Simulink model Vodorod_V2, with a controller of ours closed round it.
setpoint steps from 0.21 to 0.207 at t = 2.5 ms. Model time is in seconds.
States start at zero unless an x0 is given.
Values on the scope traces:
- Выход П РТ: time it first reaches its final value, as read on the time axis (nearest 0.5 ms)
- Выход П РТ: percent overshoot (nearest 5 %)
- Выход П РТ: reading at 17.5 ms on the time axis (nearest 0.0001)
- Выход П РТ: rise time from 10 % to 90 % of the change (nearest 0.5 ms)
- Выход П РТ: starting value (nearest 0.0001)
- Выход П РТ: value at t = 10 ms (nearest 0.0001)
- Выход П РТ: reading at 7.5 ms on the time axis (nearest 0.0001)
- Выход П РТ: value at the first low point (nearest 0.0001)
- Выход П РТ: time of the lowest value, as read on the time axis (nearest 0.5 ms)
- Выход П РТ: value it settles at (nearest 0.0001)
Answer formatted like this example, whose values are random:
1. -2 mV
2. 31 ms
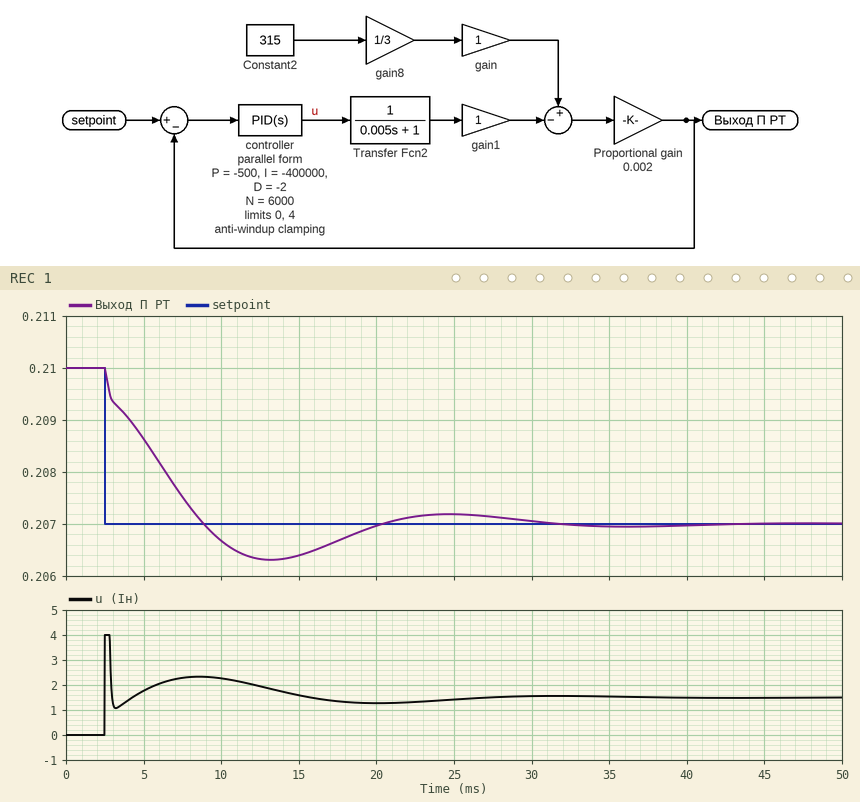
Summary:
1. 9.0 ms
2. 25 %
3. 0.2067
4. 5.5 ms
5. 0.2100
6. 0.2067
7. 0.2075
8. 0.2063
9. 13.0 ms
10. 0.2070
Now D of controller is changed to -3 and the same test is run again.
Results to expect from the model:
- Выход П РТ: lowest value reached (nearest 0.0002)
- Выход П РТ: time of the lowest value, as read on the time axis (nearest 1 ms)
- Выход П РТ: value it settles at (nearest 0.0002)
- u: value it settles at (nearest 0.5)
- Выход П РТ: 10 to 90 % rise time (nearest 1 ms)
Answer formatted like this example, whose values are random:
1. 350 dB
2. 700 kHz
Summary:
1. 0.2062
2. 14 ms
3. 0.2070
4. 1.5
5. 6 ms
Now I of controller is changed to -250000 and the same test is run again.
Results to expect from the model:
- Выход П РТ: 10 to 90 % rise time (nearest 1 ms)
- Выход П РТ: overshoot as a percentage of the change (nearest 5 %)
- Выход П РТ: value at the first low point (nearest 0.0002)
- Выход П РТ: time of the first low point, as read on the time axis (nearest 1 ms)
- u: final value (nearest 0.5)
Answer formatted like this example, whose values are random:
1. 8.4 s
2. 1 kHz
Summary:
1. 7 ms
2. 15 %
3. 0.2066
4. 16 ms
5. 1.5
